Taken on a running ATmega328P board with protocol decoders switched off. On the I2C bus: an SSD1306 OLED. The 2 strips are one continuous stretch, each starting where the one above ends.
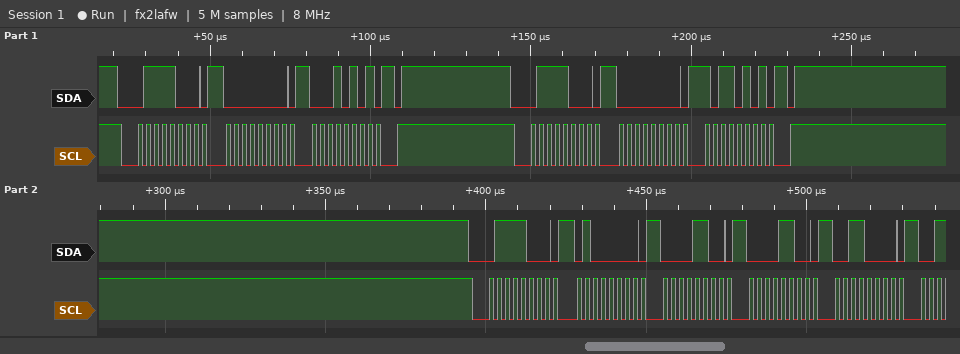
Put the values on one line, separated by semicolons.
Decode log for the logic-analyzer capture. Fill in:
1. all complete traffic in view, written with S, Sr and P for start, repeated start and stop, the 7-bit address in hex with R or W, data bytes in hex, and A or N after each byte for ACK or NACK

S 3CW A 00 A 15 A P S 3CW A 00 A B5 A P S 3CW A 40 A 0C A 0C A 30 A
